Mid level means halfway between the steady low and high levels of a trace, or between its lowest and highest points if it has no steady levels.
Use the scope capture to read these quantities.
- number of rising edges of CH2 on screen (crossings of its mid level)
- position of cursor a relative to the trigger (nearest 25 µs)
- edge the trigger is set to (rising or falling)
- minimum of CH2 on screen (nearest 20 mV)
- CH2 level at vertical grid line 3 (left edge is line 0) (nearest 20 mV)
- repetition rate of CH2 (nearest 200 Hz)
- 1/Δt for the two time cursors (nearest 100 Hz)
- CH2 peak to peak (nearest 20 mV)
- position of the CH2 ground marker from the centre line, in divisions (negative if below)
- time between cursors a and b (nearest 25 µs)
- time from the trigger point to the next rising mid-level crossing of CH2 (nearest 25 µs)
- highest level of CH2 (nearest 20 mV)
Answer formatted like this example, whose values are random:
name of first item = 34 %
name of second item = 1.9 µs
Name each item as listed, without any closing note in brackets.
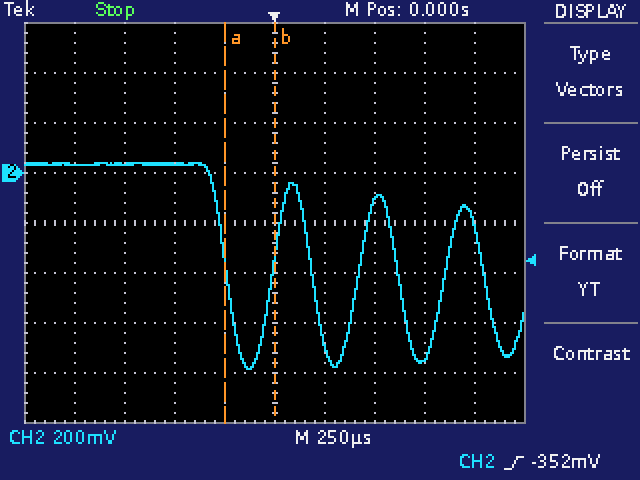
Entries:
number of rising edges of CH2 on screen = 3
position of cursor a relative to the trigger = -250 µs
edge the trigger is set to = rising
minimum of CH2 on screen = -780 mV
CH2 level at vertical grid line 3 (left edge is line 0) = 40 mV
repetition rate of CH2 = 2.4 kHz
1/Δt for the two time cursors = 4.0 kHz
CH2 peak to peak = 820 mV
position of the CH2 ground marker from the centre line, in divisions = +1.0 div
time between cursors a and b = 250 µs
time from the trigger point to the next rising mid-level crossing of CH2 = 425 µs
highest level of CH2 = 40 mV
